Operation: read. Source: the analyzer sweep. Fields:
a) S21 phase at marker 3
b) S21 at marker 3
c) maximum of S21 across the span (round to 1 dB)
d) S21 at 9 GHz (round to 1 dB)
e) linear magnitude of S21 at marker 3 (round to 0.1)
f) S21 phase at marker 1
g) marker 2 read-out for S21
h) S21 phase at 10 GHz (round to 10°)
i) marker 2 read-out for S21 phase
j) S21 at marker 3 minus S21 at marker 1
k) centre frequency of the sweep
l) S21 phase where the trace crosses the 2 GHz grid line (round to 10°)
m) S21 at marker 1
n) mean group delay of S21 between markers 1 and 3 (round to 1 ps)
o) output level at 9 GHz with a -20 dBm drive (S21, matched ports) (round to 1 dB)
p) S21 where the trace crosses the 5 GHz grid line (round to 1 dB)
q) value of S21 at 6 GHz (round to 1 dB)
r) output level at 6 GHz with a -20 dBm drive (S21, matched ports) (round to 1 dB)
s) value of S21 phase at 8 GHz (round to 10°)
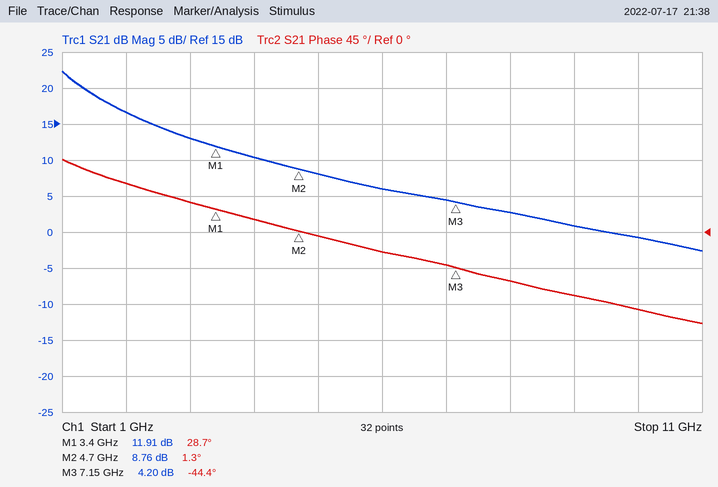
-44.4°
4.20 dB
22 dB
1 dB
1.6
28.7°
8.76 dB
-100°
1.3°
-7.71 dB
6 GHz
60°
11.91 dB
54 ps
-19 dBm
8 dB
6 dB
-14 dBm
-60°
